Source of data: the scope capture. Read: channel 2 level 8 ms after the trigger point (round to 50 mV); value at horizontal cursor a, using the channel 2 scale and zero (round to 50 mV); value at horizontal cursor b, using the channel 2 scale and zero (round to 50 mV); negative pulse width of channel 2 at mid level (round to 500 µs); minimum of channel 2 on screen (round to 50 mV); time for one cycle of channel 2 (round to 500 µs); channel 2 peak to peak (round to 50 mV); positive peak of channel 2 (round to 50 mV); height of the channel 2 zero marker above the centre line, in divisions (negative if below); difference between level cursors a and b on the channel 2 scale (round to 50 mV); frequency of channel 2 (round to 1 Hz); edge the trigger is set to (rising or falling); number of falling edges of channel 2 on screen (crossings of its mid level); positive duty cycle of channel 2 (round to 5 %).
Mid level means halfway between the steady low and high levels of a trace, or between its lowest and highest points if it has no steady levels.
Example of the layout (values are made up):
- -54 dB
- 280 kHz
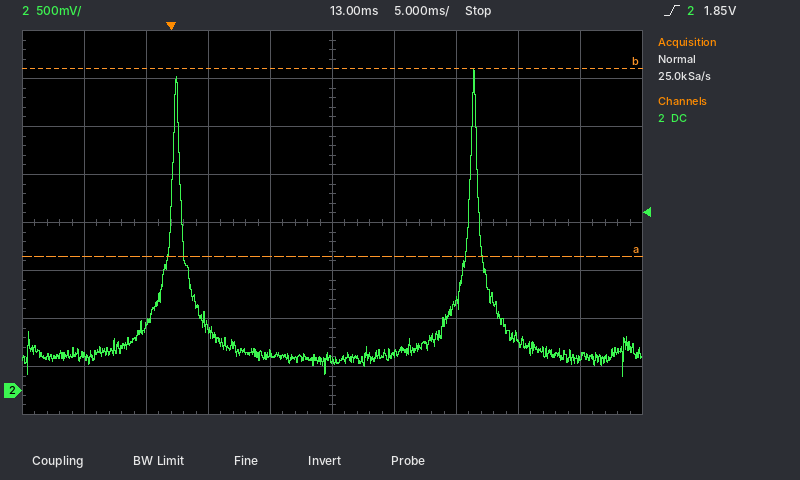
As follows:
- 400 mV
- 1.40 V
- 3.35 V
- 23.0 ms
- 150 mV
- 24.0 ms
- 3.20 V
- 3.35 V
- -3.5 div
- 1.95 V
- 42 Hz
- rising
- 2
- 5 %
